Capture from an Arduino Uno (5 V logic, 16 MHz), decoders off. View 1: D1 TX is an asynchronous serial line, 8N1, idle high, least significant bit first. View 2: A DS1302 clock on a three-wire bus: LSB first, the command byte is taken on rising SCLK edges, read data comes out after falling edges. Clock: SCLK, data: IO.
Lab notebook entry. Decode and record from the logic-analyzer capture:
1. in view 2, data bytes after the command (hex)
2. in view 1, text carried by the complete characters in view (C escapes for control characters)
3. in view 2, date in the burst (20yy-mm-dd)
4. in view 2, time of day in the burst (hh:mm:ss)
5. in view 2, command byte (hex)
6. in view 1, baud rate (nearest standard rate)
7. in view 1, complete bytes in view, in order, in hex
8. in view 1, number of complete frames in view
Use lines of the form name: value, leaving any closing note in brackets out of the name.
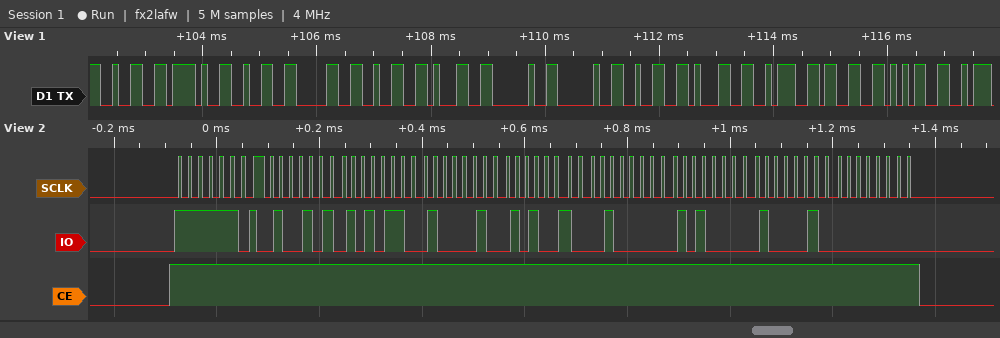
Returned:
in view 2, data bytes after the command: 52 35 21 25 02 05 21 00
in view 1, text carried by the complete characters in view: "2/2021  21:35"
in view 2, date in the burst: 2021-02-25
in view 2, time of day in the burst: 21:35:52
in view 2, command byte: 0xBF
in view 1, baud rate: 9600 baud
in view 1, complete bytes in view, in order, in hex: 0x32 0x2F 0x32 0x30 0x32 0x31 0x20 0x20 0x32 0x31 0x3A 0x33 0x35
in view 1, number of complete frames in view: 13
